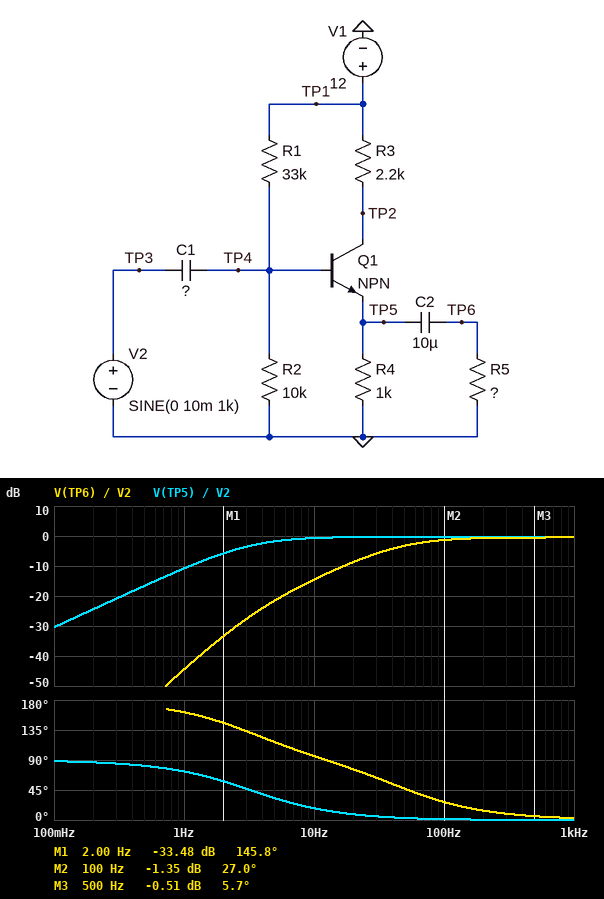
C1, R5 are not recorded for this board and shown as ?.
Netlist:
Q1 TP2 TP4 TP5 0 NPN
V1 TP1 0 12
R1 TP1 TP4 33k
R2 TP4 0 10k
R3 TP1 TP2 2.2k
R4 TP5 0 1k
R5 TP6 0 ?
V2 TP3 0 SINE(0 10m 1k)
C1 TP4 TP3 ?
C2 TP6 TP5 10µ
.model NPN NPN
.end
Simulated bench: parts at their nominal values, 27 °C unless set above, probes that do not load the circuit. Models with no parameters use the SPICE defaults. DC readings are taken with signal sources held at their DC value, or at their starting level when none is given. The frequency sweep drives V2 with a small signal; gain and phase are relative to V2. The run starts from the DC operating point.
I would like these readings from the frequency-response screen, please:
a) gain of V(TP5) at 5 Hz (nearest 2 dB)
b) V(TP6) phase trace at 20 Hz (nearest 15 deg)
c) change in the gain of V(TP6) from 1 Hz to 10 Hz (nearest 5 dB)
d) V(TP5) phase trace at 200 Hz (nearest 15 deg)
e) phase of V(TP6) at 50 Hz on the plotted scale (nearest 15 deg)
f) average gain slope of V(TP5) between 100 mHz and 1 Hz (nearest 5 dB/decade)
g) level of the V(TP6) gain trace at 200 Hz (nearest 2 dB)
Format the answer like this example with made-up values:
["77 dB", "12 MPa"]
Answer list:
["-2 dB", "75 deg", "30 dB", "0 deg", "45 deg", "20 dB/decade", "0 dB"]
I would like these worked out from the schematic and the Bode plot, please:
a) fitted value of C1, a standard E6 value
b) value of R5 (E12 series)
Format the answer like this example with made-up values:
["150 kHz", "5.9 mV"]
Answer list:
["6.8 µF", "330 Ω"]
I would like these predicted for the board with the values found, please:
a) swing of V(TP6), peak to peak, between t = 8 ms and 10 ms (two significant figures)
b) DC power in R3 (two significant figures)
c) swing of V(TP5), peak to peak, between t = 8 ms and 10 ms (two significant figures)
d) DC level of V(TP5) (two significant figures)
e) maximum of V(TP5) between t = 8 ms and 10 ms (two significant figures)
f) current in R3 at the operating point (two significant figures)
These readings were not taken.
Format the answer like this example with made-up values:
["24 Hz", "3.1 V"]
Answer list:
["19 mV", "7.5 mW", "19 mV", "1.9 V", "1.9 V", "1.8 mA"]
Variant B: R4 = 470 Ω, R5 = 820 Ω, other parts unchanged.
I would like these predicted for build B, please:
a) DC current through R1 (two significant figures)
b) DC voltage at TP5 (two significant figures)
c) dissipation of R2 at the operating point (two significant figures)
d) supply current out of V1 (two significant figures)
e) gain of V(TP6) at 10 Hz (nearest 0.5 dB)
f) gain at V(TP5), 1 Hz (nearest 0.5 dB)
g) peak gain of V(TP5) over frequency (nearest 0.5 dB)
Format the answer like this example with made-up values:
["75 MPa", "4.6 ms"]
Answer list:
["290 µA", "1.7 V", "630 µW", "3.9 mA", "-7.5 dB", "-11.5 dB", "0 dB"]
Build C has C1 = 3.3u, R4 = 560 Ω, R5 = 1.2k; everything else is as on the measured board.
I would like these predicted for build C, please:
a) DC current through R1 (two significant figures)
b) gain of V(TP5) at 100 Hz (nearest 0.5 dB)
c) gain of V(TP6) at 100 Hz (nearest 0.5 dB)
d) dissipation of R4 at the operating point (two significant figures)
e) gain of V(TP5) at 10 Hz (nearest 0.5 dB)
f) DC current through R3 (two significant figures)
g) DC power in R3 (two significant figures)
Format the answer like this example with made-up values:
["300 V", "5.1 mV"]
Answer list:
["290 µA", "0 dB", "-0.5 dB", "5.5 mW", "-2.0 dB", "3.1 mA", "21 mW"]
